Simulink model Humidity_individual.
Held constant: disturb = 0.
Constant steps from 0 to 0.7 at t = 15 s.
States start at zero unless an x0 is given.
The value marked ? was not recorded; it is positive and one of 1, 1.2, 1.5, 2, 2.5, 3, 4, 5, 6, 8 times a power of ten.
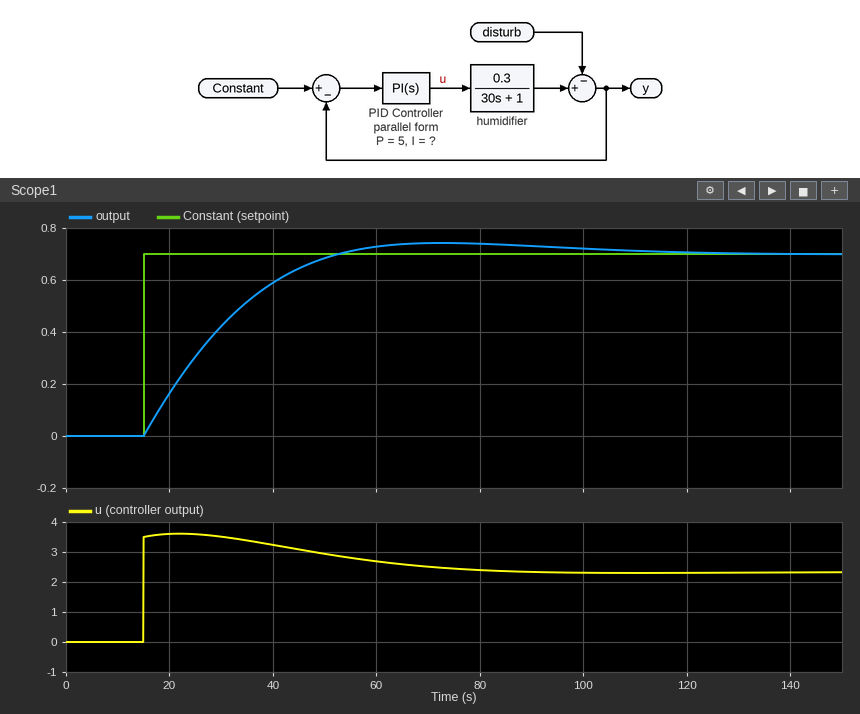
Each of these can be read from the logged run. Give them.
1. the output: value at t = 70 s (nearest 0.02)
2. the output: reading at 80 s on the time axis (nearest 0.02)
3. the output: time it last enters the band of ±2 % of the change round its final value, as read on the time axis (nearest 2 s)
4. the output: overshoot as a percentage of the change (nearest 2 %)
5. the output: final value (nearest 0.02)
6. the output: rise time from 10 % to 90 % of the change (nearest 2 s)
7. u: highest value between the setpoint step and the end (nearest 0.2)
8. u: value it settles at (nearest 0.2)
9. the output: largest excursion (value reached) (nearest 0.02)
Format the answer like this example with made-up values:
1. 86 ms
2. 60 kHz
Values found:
1. 0.74
2. 0.74
3. 108 s
4. 6 %
5. 0.70
6. 26 s
7. 3.6
8. 2.4
9. 0.74
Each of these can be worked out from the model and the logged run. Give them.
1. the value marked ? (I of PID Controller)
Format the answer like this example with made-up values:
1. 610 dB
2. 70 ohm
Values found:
1. 0.3
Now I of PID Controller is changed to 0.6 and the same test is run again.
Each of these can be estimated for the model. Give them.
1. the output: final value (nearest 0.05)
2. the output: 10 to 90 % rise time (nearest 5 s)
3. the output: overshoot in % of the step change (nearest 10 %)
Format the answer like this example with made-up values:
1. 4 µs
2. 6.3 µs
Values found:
1. 0.70
2. 15 s
3. 20 %
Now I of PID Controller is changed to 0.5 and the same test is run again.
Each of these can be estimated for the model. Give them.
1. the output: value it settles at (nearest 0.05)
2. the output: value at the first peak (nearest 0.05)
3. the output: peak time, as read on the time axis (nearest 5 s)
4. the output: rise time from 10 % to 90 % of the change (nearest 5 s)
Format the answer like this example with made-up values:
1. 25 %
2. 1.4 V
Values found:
1. 0.70
2. 0.80
3. 55 s
4. 20 s
